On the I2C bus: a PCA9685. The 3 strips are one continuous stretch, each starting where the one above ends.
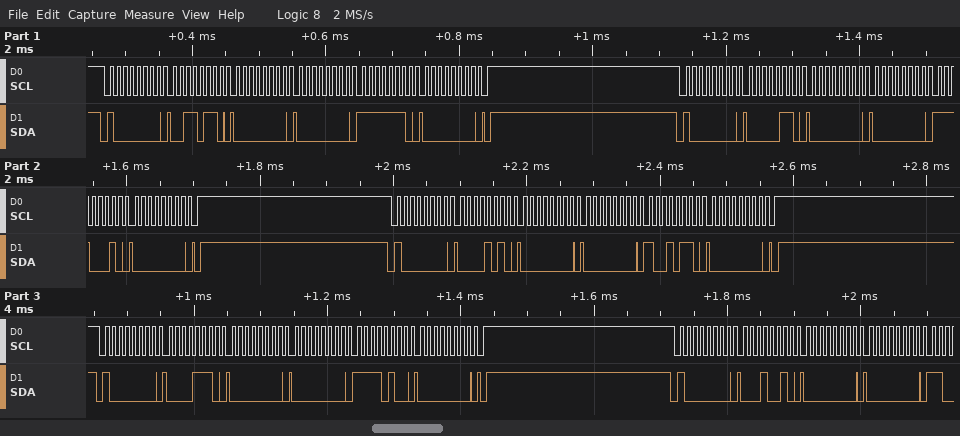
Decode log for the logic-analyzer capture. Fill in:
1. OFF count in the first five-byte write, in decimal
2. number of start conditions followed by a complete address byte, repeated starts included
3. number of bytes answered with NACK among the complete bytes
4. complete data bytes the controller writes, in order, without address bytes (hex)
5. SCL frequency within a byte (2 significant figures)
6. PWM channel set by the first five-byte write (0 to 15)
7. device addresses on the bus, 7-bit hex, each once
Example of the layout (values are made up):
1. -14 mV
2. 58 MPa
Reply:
1. 254
2. 5
3. 0
4. 36 00 00 FE 00 06 00 00 E2 00 0A 00 00 96 00 0E 00 00 F4 00 12 00 00
5. 100 kHz
6. 12
7. 0x40
